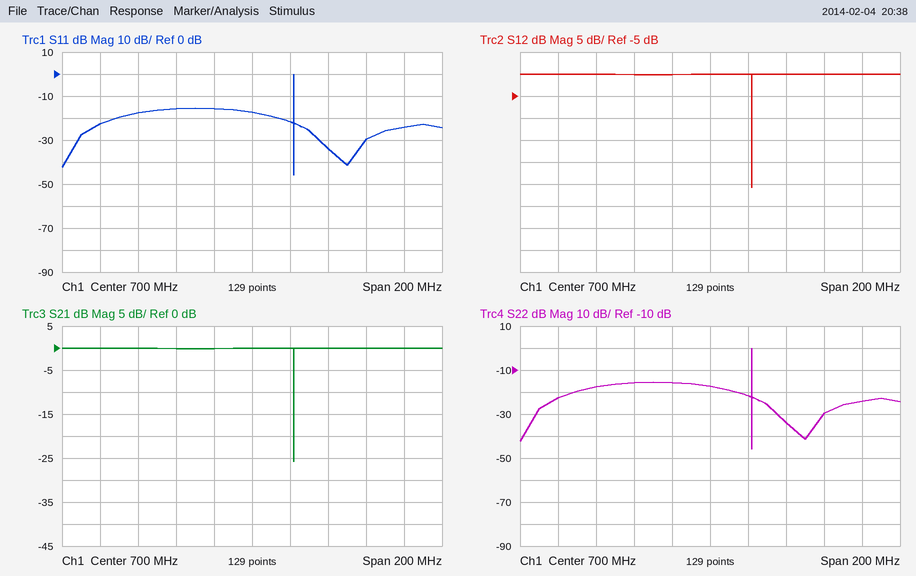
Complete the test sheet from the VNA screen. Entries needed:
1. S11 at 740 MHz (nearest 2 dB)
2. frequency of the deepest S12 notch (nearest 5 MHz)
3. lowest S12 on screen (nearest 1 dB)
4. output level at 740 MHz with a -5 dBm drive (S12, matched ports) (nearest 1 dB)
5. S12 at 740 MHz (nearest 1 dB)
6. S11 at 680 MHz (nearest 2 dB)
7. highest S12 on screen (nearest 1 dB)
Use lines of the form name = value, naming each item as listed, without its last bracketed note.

S11 at 740 MHz = -34 dB
frequency of the deepest S12 notch = 720 MHz
lowest S12 on screen = -26 dB
output level at 740 MHz with a -5 dBm drive (S12, matched ports) = -5 dBm
S12 at 740 MHz = 0 dB
S11 at 680 MHz = -16 dB
highest S12 on screen = 0 dB
